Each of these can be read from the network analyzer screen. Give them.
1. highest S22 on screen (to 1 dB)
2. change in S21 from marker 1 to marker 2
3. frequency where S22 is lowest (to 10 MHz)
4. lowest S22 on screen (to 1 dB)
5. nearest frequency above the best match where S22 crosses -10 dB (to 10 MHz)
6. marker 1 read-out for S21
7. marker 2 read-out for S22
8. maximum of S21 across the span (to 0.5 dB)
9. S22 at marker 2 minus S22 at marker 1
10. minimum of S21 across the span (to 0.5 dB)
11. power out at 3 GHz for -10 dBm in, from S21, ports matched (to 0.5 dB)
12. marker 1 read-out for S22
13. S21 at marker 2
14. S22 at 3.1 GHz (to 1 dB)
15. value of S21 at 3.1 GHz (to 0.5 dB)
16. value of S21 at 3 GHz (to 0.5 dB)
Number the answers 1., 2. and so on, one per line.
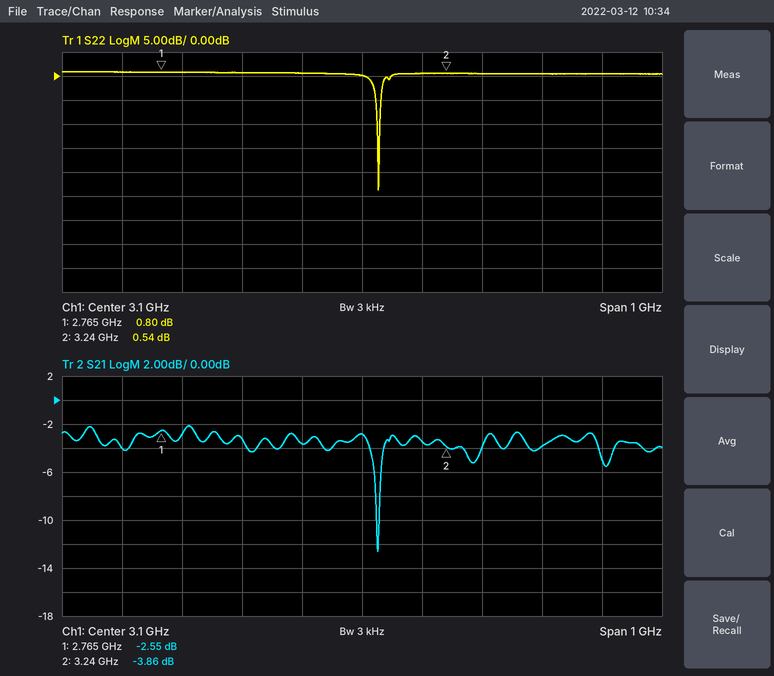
1. 1 dB
2. -1.31 dB
3. 3.13 GHz
4. -24 dB
5. 3.13 GHz
6. -2.55 dB
7. 0.54 dB
8. -2.0 dB
9. -0.26 dB
10. -12.5 dB
11. -13.5 dBm
12. 0.80 dB
13. -3.86 dB
14. 0 dB
15. -3.0 dB
16. -3.5 dB
